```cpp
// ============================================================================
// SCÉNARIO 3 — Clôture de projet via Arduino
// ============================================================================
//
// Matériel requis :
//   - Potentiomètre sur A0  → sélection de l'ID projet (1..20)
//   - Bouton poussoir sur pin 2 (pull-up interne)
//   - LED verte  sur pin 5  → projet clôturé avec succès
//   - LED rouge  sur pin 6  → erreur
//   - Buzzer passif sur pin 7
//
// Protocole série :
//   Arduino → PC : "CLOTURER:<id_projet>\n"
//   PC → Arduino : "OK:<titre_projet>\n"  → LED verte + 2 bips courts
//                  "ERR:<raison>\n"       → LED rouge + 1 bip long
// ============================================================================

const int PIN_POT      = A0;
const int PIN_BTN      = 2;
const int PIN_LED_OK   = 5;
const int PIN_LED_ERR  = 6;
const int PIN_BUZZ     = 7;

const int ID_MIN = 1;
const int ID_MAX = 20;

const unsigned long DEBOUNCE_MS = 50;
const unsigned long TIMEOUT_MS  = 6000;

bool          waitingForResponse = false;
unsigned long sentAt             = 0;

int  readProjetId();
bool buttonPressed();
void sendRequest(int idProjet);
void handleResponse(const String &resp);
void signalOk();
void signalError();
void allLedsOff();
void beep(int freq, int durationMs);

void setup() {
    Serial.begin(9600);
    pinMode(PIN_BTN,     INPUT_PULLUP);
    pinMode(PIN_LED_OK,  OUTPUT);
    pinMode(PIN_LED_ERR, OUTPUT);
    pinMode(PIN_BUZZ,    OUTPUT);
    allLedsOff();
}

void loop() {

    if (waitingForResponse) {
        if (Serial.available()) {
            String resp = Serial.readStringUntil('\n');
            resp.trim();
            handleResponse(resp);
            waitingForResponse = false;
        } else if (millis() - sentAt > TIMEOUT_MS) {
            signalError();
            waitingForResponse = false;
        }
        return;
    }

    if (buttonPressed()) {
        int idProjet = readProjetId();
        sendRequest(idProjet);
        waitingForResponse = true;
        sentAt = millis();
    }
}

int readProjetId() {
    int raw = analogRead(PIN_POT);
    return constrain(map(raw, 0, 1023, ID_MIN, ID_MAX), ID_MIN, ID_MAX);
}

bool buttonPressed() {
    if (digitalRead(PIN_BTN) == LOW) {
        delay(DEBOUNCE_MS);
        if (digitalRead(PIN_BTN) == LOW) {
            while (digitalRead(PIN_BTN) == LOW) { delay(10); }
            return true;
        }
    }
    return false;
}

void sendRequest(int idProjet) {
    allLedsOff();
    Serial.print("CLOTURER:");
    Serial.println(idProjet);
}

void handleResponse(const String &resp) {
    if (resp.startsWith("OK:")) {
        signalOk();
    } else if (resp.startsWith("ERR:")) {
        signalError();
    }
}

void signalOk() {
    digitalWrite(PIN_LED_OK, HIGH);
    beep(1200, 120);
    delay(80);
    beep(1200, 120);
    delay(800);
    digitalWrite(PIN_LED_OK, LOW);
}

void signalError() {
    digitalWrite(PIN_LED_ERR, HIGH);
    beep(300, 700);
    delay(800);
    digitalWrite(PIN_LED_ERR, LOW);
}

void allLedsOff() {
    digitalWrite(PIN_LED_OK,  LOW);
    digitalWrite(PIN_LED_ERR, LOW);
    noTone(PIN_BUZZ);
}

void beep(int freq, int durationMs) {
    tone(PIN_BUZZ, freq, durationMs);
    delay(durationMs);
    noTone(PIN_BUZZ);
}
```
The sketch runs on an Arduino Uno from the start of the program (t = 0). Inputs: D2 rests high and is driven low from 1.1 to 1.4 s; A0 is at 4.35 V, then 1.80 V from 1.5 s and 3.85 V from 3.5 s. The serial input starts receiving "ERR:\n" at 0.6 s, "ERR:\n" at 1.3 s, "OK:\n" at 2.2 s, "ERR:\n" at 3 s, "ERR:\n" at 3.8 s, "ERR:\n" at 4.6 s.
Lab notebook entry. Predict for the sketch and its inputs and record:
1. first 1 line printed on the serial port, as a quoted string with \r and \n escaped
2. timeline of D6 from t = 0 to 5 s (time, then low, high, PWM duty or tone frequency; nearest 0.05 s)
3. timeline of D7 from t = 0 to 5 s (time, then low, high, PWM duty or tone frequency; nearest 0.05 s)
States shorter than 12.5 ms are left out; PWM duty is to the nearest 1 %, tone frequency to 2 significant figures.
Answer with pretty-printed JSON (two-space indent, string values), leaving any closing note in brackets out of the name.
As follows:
{
  "first 1 line printed on the serial port, as a quoted string with \\r and \\n escaped": "\"CLOTURER:17\\r\\n\"",
  "timeline of D6 from t = 0 to 5 s": "0 s low; 1.4 s high; 2.9 s low",
  "timeline of D7 from t = 0 to 5 s": "0 s low; 1.4 s tone 300 Hz; 2.1 s low"
}
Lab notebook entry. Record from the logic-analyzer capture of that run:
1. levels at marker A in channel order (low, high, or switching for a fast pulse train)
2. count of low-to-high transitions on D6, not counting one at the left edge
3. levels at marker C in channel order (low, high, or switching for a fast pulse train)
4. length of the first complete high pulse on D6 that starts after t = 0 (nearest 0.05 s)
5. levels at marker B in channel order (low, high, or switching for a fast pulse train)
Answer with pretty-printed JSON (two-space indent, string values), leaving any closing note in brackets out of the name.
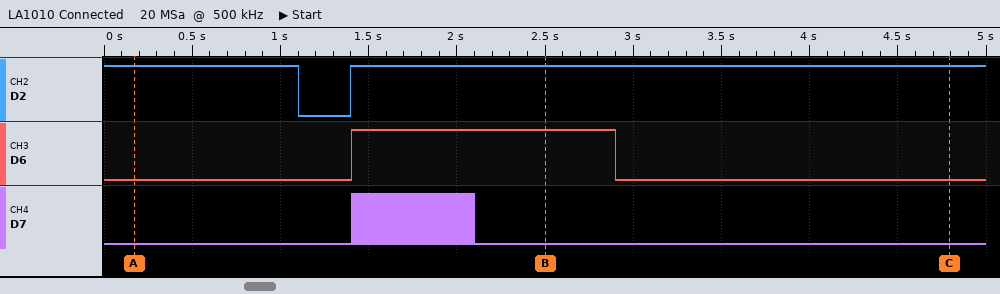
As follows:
{
  "levels at marker A in channel order": "D2 high, D6 low, D7 low",
  "count of low-to-high transitions on D6, not counting one at the left edge": "1",
  "levels at marker C in channel order": "D2 high, D6 low, D7 low",
  "length of the first complete high pulse on D6 that starts after t = 0": "1.50 s",
  "levels at marker B in channel order": "D2 high, D6 high, D7 low"
}
